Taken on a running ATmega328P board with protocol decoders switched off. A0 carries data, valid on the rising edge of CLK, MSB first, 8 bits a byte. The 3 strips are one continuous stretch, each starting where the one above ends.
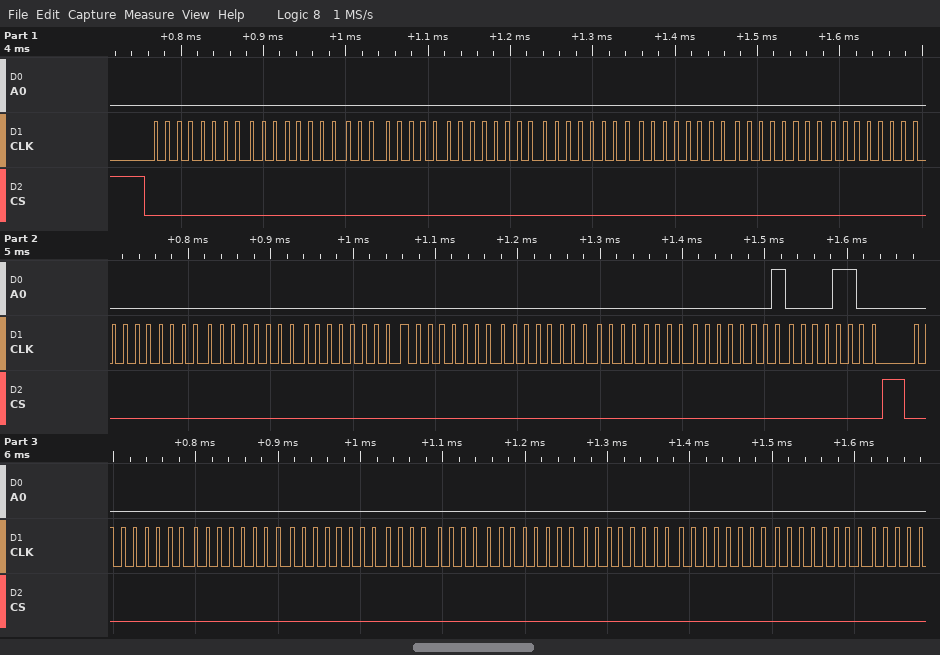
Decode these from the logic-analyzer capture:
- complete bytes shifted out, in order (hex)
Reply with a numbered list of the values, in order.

1. 0x00 0x00 0x00 0x00 0x00 0x00 0x00 0x00 0x00 0x00 0x00 0x00 0x00 0x00 0x01 0x0C 0x00 0x00 0x00 0x00 0x00 0x00 0x00 0x00
